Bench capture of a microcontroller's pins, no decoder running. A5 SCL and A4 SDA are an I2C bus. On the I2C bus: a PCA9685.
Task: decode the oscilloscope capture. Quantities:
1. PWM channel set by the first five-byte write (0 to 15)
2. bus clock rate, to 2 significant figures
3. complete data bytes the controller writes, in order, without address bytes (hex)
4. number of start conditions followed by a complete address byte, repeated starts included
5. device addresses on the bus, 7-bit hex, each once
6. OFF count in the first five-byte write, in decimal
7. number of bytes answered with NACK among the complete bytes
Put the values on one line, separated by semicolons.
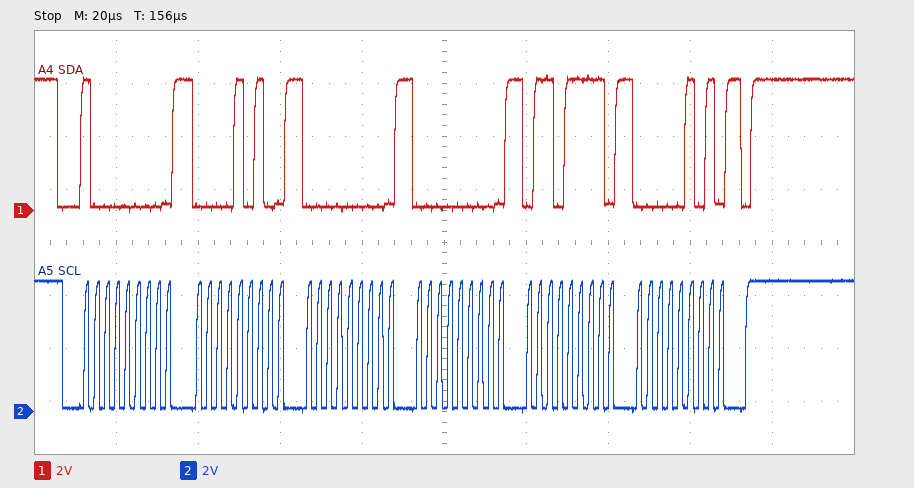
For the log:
1; 400 kHz; 0A 00 00 6F 05; 1; 0x40; 1391; 0
